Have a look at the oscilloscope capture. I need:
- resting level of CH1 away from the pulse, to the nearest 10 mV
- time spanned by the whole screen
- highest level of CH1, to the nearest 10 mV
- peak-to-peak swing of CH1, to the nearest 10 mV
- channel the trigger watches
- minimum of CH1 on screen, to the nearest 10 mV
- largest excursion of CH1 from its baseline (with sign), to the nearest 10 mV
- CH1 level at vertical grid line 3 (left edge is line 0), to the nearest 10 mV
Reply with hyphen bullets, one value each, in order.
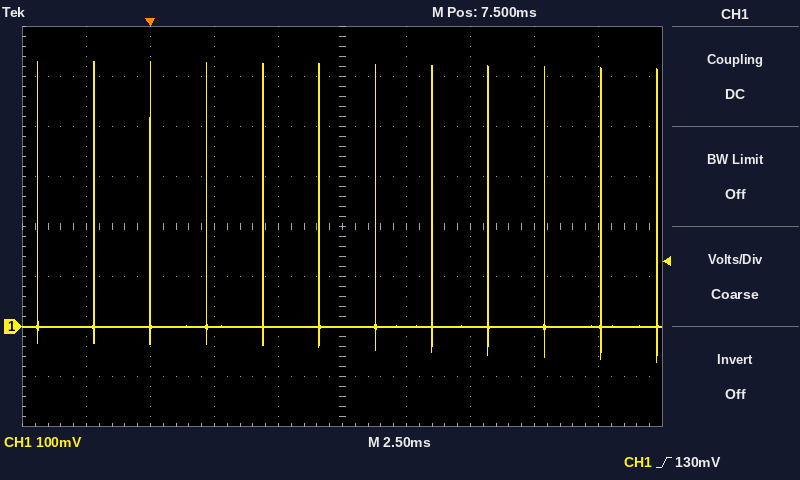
- 0 mV
- 25 ms
- 530 mV
- 600 mV
- CH1
- -70 mV
- +530 mV
- 0 mV
